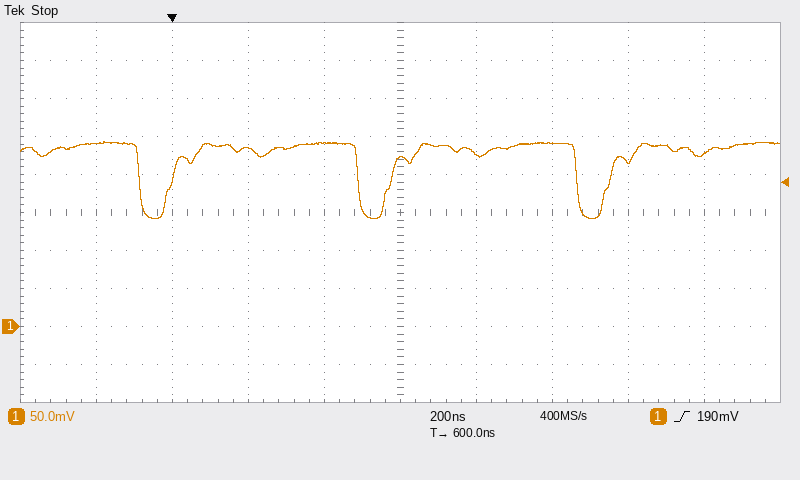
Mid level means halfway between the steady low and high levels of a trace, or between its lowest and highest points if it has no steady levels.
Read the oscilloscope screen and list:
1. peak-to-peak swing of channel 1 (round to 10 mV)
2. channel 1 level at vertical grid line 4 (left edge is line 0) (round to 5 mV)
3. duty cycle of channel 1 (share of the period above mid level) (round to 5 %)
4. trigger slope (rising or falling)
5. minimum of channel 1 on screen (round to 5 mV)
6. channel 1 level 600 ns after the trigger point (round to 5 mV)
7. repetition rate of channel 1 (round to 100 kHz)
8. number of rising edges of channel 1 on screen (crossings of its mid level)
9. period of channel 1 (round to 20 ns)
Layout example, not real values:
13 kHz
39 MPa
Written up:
100 mV
240 mV
85 %
rising
140 mV
220 mV
1.7 MHz
3
580 ns
